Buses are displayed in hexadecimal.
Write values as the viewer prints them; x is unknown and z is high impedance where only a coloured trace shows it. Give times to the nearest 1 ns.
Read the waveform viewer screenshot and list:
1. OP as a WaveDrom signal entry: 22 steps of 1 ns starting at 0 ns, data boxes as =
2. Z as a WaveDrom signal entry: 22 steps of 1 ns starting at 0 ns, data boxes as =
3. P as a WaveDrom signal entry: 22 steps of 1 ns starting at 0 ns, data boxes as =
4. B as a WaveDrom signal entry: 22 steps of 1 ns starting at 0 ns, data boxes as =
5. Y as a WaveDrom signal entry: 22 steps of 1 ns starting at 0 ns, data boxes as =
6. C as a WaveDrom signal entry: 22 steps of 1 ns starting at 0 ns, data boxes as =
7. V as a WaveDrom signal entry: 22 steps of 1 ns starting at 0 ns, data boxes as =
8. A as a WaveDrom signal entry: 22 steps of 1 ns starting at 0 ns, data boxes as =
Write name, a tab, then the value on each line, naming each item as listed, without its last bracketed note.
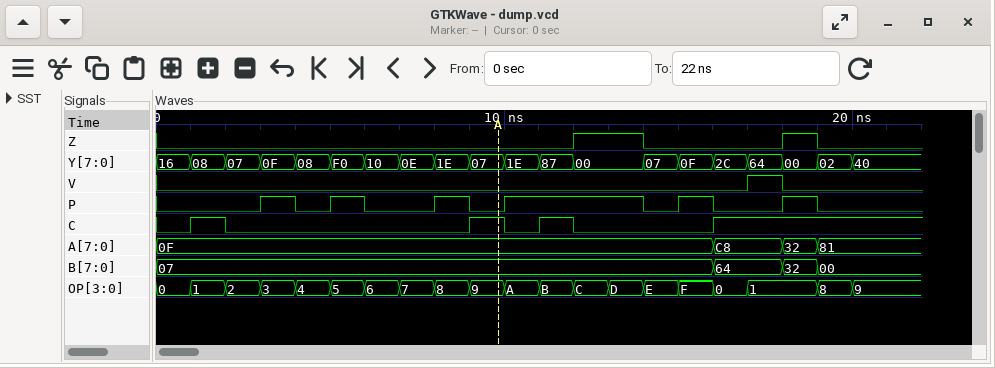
OP as a WaveDrom signal entry: 22 steps of 1 ns starting at 0 ns, data boxes as =	{name: 'OP', wave: '==================.==.', data: '0 1 2 3 4 5 6 7 8 9 A B C D E F 0 1 8 9'}
Z as a WaveDrom signal entry: 22 steps of 1 ns starting at 0 ns, data boxes as =	{name: 'Z', wave: '0...........1.0...10..'}
P as a WaveDrom signal entry: 22 steps of 1 ns starting at 0 ns, data boxes as =	{name: 'P', wave: '0..1010.101...010.10..'}
B as a WaveDrom signal entry: 22 steps of 1 ns starting at 0 ns, data boxes as =	{name: 'B', wave: '=...............=.==..', data: '07 64 32 00'}
Y as a WaveDrom signal entry: 22 steps of 1 ns starting at 0 ns, data boxes as =	{name: 'Y', wave: '=============.=======.', data: '16 08 07 0F 08 F0 10 0E 1E 07 1E 87 00 07 0F 2C 64 00 02 40'}
C as a WaveDrom signal entry: 22 steps of 1 ns starting at 0 ns, data boxes as =	{name: 'C', wave: '010......1010...1.....'}
V as a WaveDrom signal entry: 22 steps of 1 ns starting at 0 ns, data boxes as =	{name: 'V', wave: '0................10...'}
A as a WaveDrom signal entry: 22 steps of 1 ns starting at 0 ns, data boxes as =	{name: 'A', wave: '=...............=.==..', data: '0F C8 32 81'}
